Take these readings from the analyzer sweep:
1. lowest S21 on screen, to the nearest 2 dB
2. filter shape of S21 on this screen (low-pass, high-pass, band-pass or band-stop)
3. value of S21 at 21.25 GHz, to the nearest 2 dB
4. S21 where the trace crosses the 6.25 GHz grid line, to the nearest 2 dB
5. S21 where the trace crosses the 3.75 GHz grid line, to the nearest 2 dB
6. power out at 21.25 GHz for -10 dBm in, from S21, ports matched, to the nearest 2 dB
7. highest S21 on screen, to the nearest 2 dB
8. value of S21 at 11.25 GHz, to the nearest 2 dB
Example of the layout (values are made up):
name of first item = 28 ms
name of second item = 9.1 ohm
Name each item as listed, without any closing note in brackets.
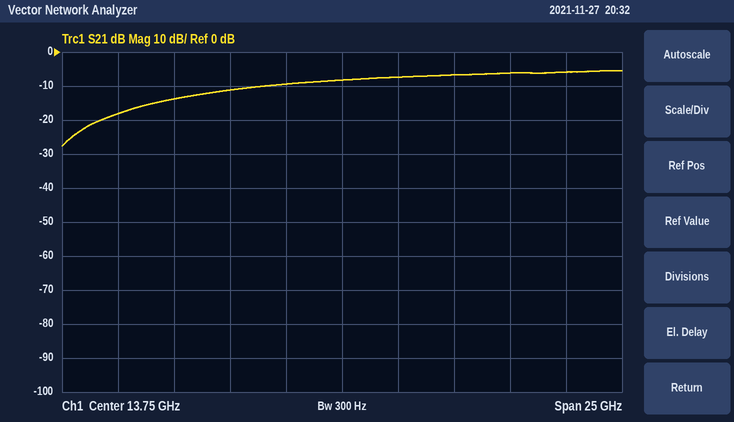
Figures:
lowest S21 on screen, to the nearest 2 dB = -28 dB
filter shape of S21 on this screen = high-pass
value of S21 at 21.25 GHz, to the nearest 2 dB = -6 dB
S21 where the trace crosses the 6.25 GHz grid line, to the nearest 2 dB = -14 dB
S21 where the trace crosses the 3.75 GHz grid line, to the nearest 2 dB = -18 dB
power out at 21.25 GHz for -10 dBm in, from S21, ports matched, to the nearest 2 dB = -16 dBm
highest S21 on screen, to the nearest 2 dB = -6 dB
value of S21 at 11.25 GHz, to the nearest 2 dB = -10 dB
